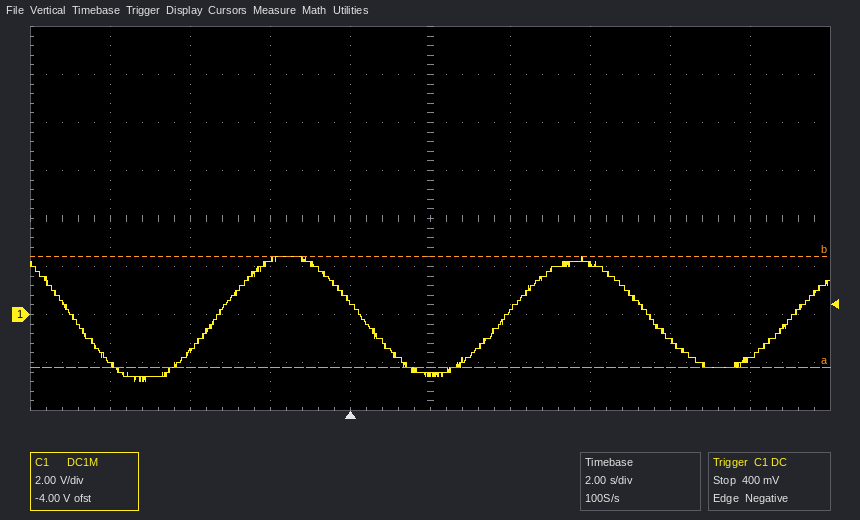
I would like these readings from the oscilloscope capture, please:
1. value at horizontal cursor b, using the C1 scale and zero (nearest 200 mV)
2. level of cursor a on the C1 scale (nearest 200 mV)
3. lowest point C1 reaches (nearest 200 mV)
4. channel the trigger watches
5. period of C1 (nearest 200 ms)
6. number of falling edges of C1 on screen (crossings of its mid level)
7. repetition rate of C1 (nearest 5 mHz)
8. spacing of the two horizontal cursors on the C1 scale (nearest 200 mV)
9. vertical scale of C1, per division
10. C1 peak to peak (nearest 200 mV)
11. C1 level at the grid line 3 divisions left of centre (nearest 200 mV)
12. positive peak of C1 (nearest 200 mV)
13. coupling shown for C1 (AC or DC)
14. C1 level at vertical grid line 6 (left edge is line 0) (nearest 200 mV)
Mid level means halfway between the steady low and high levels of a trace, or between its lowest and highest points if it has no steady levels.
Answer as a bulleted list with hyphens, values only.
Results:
- 2.4 V
- -2.2 V
- -2.8 V
- C1
- 7.2 s
- 3
- 140 mHz
- 4.6 V
- 2 V
- 5.2 V
- -1.6 V
- 2.4 V
- DC
- 200 mV
